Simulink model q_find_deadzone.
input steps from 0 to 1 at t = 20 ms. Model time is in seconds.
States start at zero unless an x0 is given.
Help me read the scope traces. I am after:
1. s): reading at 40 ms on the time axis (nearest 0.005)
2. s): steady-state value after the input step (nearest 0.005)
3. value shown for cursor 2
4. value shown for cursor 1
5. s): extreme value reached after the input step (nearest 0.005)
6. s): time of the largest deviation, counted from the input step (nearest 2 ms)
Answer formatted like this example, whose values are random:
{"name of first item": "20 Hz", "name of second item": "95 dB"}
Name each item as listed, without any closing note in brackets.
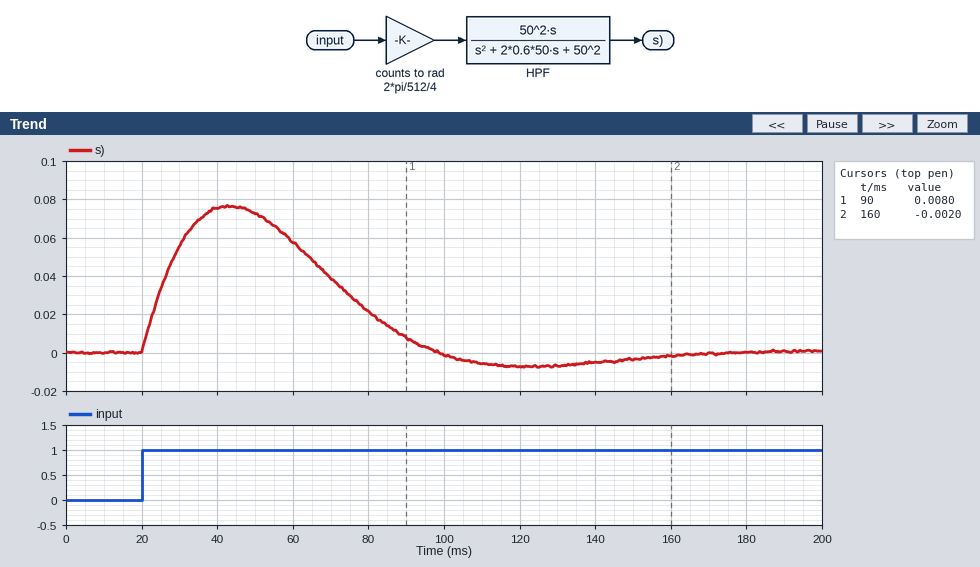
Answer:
{"s): reading at 40 ms on the time axis": "0.075", "s): steady-state value after the input step": "0.000", "value shown for cursor 2": "-0.0020", "value shown for cursor 1": "0.0080", "s): extreme value reached after the input step": "0.075", "s): time of the largest deviation, counted from the input step": "24 ms"}
